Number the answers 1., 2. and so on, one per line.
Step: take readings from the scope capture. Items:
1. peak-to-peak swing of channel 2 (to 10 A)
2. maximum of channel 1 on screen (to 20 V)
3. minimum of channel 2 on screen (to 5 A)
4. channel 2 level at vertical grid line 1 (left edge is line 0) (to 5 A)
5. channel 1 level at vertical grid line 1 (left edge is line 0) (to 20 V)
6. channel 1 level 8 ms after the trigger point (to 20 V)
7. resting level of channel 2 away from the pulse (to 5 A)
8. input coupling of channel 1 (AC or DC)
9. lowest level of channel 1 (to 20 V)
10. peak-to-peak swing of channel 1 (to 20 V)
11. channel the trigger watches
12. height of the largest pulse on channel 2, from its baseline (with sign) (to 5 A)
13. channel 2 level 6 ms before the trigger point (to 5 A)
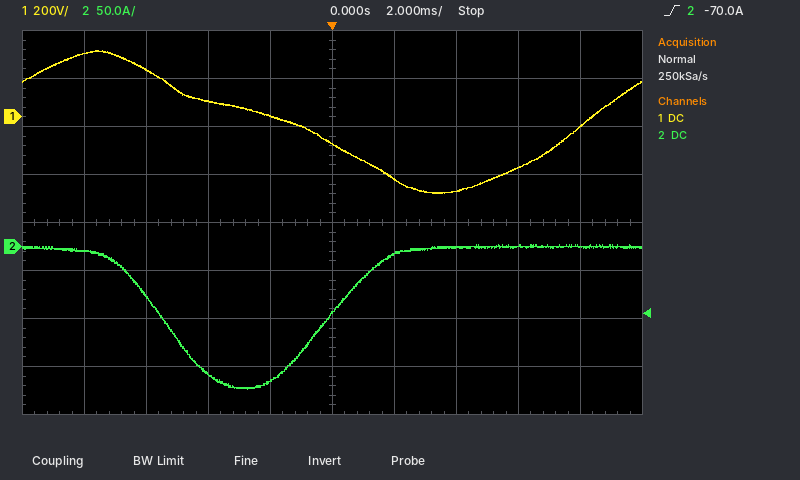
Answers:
1. 150 A
2. 280 V
3. -150 A
4. -5 A
5. 260 V
6. -40 V
7. 0 A
8. DC
9. -320 V
10. 600 V
11. channel 2
12. -150 A
13. -50 A
